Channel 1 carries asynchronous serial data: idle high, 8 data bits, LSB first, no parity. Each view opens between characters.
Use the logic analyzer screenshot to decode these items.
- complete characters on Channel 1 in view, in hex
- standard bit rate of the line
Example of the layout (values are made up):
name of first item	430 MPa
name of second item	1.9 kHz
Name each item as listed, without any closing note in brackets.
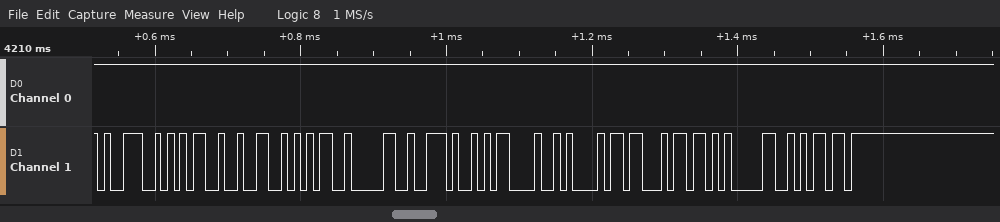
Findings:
complete characters on Channel 1 in view, in hex	39, 35, 32, 35, 30, 2E, 0D, 0A, 1B, 5B, 30, 6D
standard bit rate of the line	115200 baud
